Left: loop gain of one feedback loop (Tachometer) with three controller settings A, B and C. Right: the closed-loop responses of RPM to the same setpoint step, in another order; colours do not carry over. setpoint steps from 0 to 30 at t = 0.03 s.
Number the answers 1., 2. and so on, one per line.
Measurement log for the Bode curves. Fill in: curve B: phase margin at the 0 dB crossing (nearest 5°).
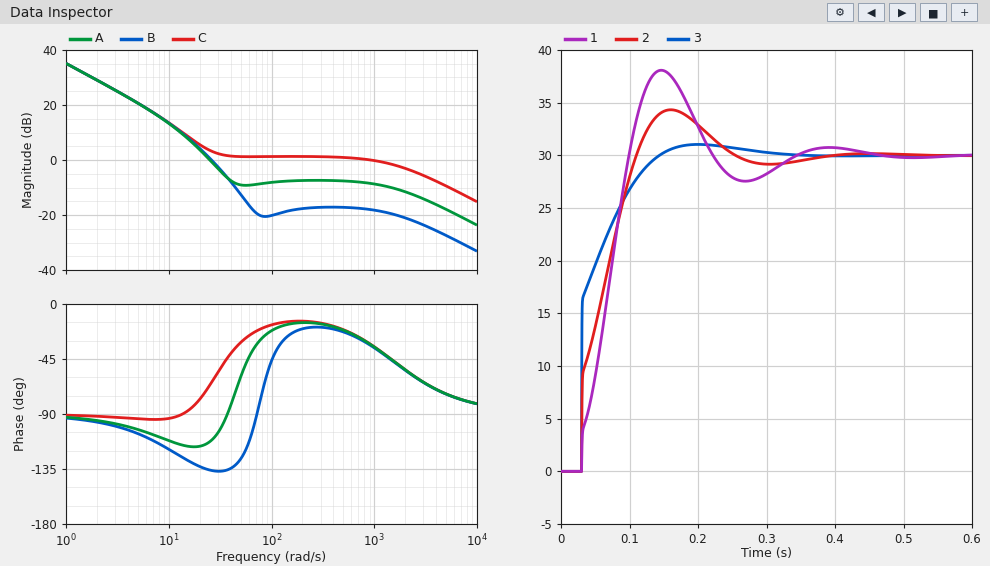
1. 45°
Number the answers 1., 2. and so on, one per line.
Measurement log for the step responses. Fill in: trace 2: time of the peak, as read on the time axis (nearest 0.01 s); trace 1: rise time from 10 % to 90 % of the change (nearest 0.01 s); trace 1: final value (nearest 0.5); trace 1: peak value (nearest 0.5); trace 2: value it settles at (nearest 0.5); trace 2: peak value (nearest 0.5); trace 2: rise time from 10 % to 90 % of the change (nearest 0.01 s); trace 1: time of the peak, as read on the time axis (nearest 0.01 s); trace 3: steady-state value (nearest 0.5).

1. 0.16 s
2. 0.06 s
3. 30.0
4. 38.0
5. 30.0
6. 34.5
7. 0.07 s
8. 0.15 s
9. 30.0
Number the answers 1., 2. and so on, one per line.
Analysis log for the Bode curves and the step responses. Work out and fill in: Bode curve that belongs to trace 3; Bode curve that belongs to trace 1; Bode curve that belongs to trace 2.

1. C
2. B
3. A
